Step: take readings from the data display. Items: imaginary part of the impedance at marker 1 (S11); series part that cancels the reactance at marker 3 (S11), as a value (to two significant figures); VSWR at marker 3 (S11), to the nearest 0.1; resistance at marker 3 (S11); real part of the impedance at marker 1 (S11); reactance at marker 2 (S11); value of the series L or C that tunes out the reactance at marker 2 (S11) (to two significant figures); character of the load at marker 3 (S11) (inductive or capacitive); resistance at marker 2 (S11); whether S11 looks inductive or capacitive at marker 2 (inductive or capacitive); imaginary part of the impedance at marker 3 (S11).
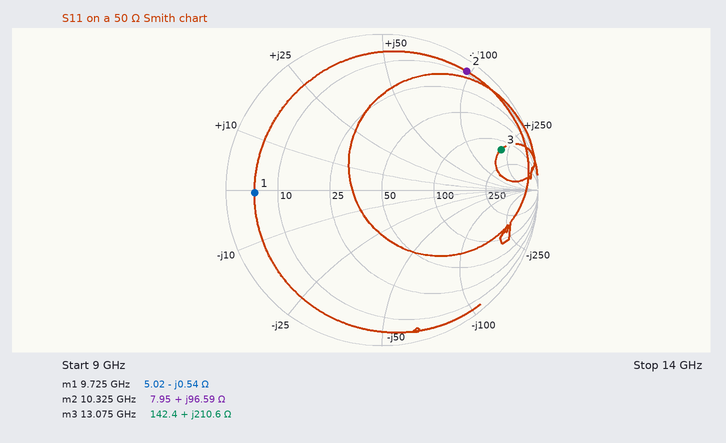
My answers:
-0.54 Ω
58 fF
9.3
142.4 Ω
5.02 Ω
+96.59 Ω
160 fF
inductive
7.95 Ω
inductive
+210.6 Ω
